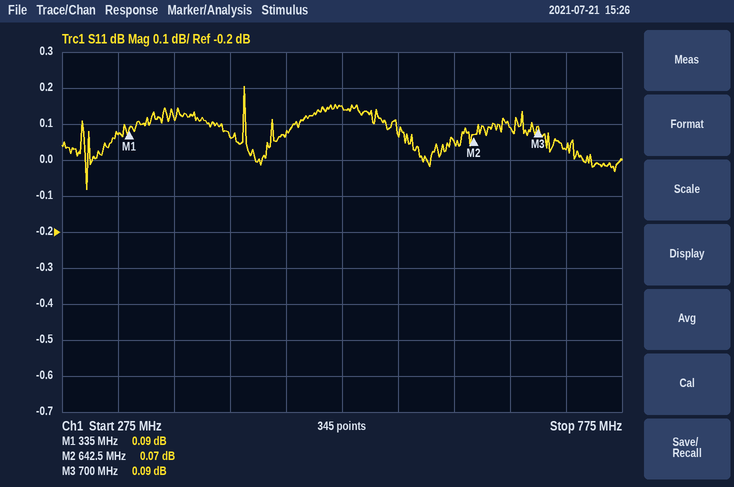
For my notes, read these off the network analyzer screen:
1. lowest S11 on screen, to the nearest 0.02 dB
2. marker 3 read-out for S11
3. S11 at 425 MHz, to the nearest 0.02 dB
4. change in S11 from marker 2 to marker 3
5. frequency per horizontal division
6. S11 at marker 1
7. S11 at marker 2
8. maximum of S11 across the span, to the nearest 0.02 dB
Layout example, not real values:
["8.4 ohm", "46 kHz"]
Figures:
["-0.08 dB", "0.09 dB", "0.06 dB", "0.02 dB", "50 MHz", "0.09 dB", "0.07 dB", "0.20 dB"]
